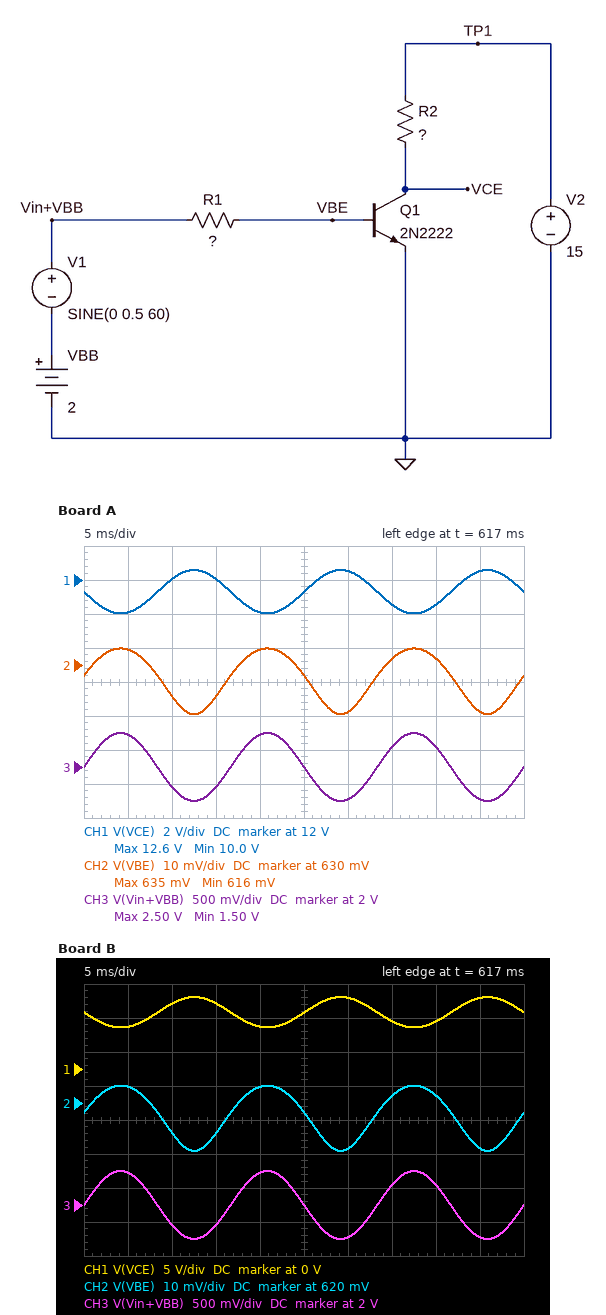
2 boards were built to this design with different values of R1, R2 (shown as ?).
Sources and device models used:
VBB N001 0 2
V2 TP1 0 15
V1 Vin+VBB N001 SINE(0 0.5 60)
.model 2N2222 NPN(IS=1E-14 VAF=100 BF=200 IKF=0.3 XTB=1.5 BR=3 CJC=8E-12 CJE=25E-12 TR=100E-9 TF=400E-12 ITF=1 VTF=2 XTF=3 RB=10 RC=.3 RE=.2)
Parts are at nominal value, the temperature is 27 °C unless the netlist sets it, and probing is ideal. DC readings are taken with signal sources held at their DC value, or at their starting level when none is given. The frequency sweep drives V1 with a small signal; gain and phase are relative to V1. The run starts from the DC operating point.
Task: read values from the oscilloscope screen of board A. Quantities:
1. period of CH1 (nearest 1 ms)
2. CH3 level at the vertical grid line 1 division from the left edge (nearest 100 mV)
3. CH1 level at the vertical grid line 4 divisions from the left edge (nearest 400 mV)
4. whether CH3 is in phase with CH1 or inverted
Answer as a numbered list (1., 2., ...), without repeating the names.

1. 17 ms
2. 2.5 V
3. 10.0 V
4. inverted
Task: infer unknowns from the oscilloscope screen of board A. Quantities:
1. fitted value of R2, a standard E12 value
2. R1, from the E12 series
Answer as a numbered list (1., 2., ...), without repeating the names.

1. 10 kΩ
2. 820 kΩ
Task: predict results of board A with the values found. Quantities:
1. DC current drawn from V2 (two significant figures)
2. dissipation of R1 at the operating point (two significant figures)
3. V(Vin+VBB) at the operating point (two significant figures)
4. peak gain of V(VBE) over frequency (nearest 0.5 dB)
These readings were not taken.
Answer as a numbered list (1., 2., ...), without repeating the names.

1. 370 µA
2. 2.3 µW
3. 2.0 V
4. -34.5 dB
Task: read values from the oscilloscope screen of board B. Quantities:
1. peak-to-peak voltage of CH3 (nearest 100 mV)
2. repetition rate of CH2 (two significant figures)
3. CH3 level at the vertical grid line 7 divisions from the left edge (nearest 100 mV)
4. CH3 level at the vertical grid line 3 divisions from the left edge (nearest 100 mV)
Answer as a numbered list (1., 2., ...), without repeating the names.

1. 1.0 V
2. 60 Hz
3. 2.3 V
4. 1.7 V
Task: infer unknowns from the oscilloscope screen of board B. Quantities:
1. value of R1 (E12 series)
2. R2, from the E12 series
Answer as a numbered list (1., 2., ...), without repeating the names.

1. 1.2 MΩ
2. 27 kΩ
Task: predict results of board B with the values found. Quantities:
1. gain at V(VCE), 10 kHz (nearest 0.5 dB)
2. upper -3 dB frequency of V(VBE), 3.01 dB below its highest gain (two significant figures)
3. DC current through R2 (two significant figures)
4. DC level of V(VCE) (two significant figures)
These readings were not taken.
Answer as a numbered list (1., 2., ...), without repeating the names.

1. 9.0 dB
2. 7.8 kHz
3. 250 µA
4. 8.3 V
